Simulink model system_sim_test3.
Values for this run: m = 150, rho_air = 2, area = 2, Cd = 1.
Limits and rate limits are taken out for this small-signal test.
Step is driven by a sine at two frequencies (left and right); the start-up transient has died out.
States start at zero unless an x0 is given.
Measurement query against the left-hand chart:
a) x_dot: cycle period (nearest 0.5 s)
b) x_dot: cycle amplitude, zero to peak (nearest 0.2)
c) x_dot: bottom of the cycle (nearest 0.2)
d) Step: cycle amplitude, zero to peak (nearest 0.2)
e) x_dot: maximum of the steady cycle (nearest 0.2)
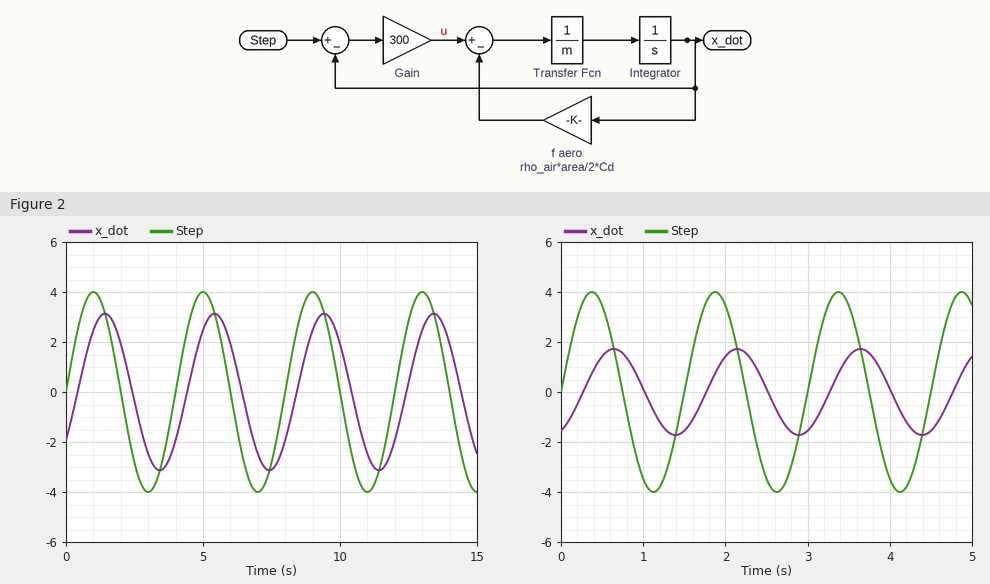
4.0 s
3.2
-3.2
4.0
3.2
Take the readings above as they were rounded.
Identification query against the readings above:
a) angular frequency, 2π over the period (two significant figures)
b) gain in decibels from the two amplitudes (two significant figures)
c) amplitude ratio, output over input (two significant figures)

1.6 rad/s
-1.9 dB
0.80
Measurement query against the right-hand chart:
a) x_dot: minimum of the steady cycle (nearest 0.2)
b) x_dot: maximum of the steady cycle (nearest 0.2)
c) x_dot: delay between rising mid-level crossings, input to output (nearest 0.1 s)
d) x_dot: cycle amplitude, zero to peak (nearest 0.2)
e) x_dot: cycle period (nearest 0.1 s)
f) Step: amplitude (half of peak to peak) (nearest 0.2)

-1.8
1.8
0.3 s
1.8
1.5 s
4.0
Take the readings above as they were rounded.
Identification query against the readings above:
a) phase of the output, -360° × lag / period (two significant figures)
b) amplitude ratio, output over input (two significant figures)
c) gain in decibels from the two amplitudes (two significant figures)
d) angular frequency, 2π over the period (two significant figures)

-72°
0.45
-6.9 dB
4.2 rad/s
